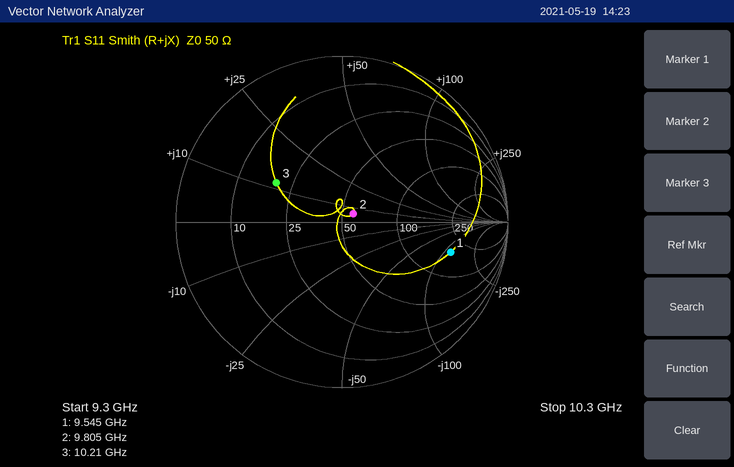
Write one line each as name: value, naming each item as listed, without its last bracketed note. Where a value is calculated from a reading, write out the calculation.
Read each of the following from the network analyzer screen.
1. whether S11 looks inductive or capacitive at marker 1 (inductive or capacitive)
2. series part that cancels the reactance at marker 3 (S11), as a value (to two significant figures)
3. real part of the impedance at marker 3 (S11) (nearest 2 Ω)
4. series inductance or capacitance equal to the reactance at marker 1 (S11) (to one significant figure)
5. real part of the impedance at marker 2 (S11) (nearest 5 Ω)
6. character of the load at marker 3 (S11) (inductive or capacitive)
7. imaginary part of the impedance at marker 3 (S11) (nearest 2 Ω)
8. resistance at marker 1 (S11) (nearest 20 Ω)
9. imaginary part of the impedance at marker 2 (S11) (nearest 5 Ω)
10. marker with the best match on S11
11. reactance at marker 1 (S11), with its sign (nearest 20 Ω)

whether S11 looks inductive or capacitive at marker 1: capacitive
series part that cancels the reactance at marker 3 (S11), as a value: C = 1/(2π × 10.21 GHz × 12 Ω) ≈ 1.3 pF
real part of the impedance at marker 3 (S11): 20 Ω
series inductance or capacitance equal to the reactance at marker 1 (S11): C = 1/(2π × 9.545 GHz × 120 Ω) ≈ 139 fF, so 100 fF to one significant figure
real part of the impedance at marker 2 (S11): 55 Ω
character of the load at marker 3 (S11): inductive
imaginary part of the impedance at marker 3 (S11): +12 Ω
resistance at marker 1 (S11): 180 Ω
imaginary part of the impedance at marker 2 (S11): +5 Ω
marker with the best match on S11: marker 2
reactance at marker 1 (S11), with its sign: -120 Ω
